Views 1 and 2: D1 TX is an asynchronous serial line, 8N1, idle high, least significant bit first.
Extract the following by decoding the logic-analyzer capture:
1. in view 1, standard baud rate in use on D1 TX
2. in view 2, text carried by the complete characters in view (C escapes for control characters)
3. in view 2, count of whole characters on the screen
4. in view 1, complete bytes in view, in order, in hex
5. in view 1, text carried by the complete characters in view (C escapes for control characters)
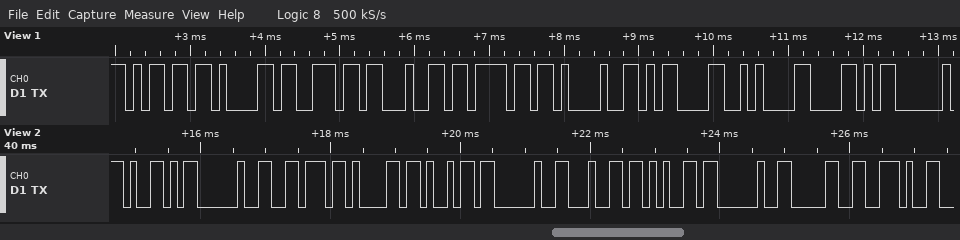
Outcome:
9600 baud
"Y vai de 0."
11
6D 61 6E 64 6F 21 0D 0A 58
"mando!\r\nX"
